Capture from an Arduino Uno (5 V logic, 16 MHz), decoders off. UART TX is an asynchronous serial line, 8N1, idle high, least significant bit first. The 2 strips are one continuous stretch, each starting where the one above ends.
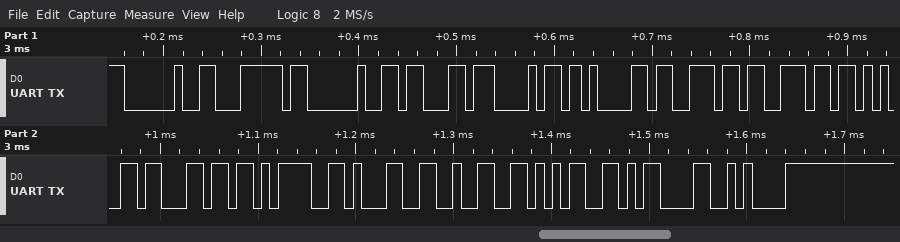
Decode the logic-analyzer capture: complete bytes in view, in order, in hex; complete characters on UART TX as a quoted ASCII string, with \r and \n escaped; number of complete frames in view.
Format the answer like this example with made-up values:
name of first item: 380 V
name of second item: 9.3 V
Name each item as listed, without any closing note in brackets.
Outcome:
complete bytes in view, in order, in hex: 20 7C 20 63 68 61 6E 6E 65 6C 3D 31 32 35 0D 0A
complete characters on UART TX as a quoted ASCII string, with \r and \n escaped: " | channel=125\r\n"
number of complete frames in view: 16
